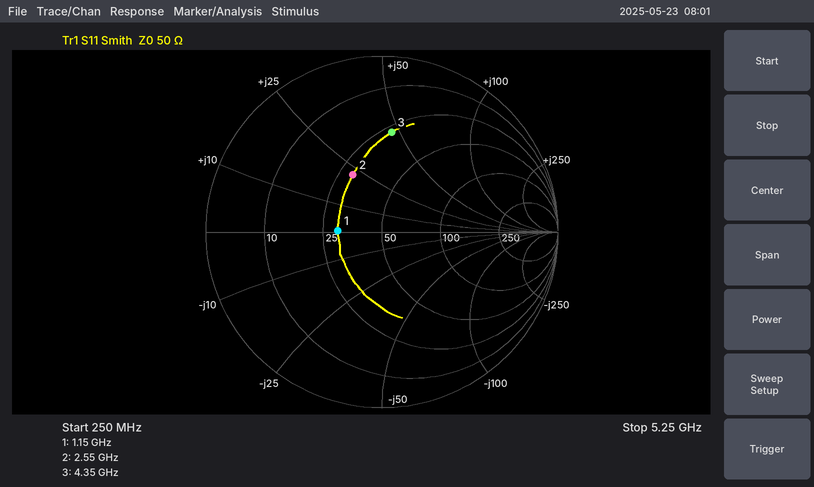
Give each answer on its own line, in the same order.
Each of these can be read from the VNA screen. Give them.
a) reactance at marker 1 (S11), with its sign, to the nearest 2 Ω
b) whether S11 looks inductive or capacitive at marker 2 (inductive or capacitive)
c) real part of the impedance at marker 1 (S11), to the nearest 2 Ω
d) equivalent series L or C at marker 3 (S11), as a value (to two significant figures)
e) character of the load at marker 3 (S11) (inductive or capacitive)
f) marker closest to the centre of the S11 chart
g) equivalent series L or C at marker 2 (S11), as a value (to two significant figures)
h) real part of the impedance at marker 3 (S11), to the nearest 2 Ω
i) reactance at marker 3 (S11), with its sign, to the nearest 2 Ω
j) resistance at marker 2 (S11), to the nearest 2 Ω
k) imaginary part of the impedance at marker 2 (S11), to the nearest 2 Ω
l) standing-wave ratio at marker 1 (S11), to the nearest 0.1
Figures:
0 Ω
inductive
30 Ω
1.7 nH
inductive
marker 1
1.4 nH
28 Ω
+46 Ω
30 Ω
+22 Ω
1.7
